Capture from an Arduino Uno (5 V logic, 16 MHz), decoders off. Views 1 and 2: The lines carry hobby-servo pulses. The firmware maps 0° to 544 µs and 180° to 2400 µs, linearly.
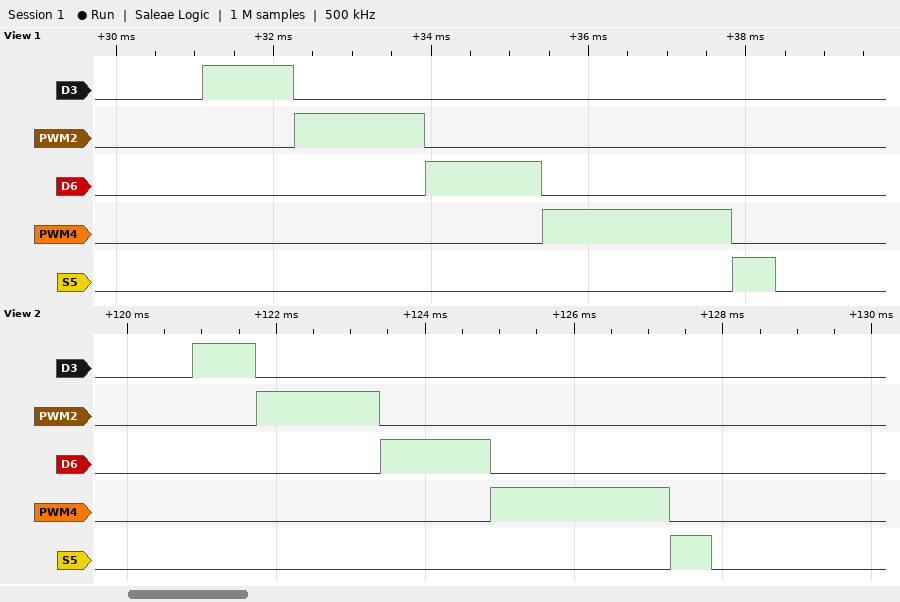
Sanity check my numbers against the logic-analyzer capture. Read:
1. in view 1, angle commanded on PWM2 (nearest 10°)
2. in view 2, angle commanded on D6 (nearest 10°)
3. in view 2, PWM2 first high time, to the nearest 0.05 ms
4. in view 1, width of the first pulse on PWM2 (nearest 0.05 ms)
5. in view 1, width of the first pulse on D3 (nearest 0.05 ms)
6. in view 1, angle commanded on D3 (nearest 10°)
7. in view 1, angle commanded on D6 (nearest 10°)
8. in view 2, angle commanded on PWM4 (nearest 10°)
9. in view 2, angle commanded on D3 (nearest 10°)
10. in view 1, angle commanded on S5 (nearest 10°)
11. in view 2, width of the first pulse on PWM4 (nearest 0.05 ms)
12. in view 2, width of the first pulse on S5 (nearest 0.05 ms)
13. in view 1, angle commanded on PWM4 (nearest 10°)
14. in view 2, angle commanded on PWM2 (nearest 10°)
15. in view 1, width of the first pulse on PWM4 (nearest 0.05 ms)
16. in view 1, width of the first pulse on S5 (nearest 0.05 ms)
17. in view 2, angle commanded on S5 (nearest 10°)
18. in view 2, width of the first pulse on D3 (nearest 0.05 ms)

110°
90°
1.65 ms
1.65 ms
1.15 ms
60°
90°
180°
30°
0°
2.40 ms
0.55 ms
180°
110°
2.40 ms
0.55 ms
0°
0.85 ms
